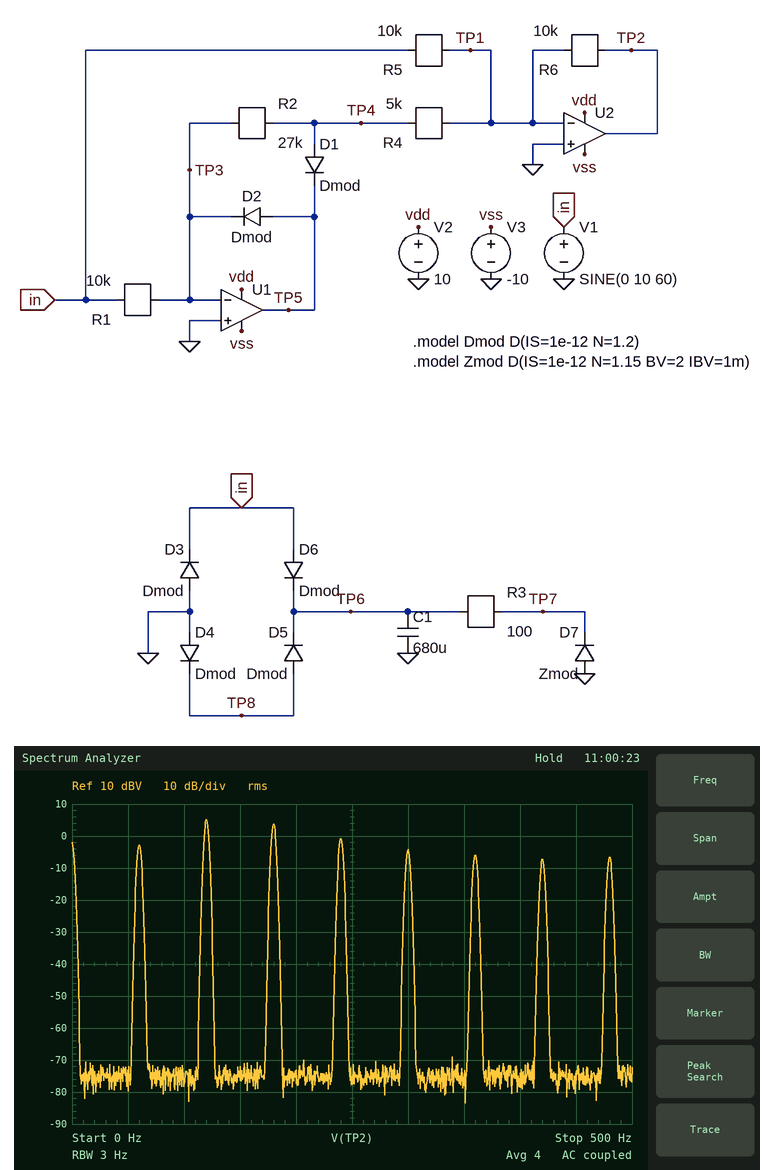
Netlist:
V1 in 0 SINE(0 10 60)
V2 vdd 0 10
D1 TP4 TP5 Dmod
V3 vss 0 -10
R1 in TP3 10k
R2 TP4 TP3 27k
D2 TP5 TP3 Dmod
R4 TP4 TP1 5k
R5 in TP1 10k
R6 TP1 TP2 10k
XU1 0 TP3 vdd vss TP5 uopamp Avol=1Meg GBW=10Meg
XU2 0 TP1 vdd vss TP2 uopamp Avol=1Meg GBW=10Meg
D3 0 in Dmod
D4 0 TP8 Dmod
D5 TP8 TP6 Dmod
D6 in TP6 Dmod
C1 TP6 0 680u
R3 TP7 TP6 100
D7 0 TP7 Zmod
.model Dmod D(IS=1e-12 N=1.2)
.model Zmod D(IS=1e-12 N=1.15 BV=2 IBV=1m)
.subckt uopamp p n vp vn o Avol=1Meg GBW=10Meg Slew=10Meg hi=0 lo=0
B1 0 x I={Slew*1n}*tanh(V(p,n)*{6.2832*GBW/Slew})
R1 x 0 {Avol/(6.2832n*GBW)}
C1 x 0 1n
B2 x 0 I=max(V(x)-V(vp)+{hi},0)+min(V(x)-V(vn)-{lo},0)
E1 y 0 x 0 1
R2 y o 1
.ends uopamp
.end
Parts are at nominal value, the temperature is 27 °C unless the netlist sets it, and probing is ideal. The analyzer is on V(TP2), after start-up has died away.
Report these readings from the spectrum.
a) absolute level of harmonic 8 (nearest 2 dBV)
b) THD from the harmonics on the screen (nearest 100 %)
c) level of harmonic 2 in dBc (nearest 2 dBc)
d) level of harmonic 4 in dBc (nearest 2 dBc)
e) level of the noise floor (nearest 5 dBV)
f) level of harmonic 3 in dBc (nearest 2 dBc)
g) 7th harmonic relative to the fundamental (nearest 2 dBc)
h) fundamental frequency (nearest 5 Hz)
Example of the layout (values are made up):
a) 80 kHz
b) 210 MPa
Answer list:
a) -6 dBV
b) 400 %
c) 8 dBc
d) 2 dBc
e) -75 dBV
f) 6 dBc
g) -4 dBc
h) 60 Hz
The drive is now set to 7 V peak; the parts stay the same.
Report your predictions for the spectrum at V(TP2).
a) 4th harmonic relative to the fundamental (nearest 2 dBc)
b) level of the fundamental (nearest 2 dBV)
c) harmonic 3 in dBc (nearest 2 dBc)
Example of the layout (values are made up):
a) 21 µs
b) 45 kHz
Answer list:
a) -8 dBc
b) 6 dBV
c) -4 dBc
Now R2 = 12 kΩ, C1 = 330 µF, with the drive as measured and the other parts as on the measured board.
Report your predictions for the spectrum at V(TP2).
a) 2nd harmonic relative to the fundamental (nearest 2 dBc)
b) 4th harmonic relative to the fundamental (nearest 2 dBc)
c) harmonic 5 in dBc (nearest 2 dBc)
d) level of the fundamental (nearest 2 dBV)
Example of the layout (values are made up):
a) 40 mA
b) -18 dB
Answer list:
a) 18 dBc
b) 10 dBc
c) -4 dBc
d) -10 dBV
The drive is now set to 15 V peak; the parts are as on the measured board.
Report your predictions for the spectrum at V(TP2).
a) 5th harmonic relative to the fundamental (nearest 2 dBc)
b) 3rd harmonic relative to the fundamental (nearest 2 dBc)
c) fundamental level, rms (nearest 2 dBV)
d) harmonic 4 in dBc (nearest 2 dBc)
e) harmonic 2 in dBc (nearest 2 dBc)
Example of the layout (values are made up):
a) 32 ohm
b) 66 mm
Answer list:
a) -2 dBc
b) 2 dBc
c) 2 dBV
d) 0 dBc
e) -10 dBc
